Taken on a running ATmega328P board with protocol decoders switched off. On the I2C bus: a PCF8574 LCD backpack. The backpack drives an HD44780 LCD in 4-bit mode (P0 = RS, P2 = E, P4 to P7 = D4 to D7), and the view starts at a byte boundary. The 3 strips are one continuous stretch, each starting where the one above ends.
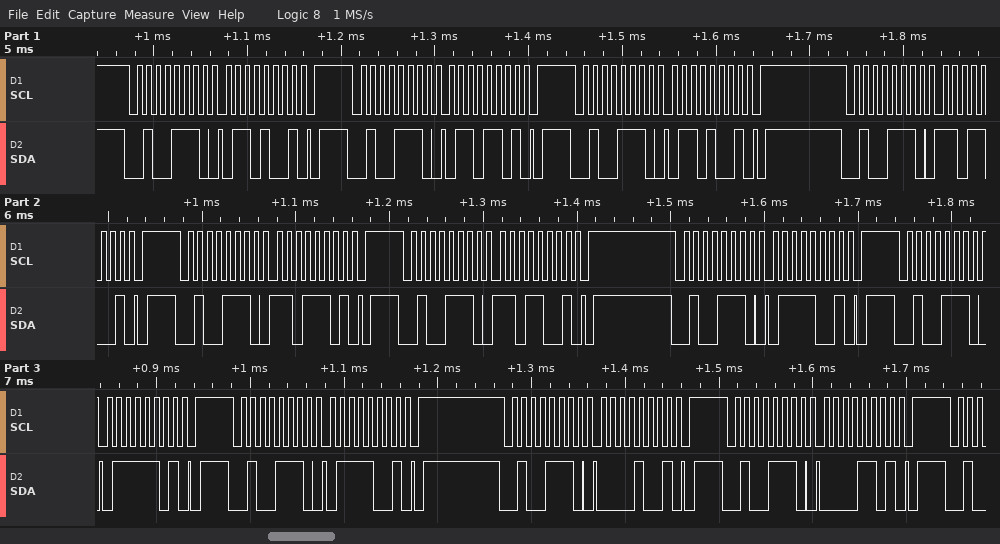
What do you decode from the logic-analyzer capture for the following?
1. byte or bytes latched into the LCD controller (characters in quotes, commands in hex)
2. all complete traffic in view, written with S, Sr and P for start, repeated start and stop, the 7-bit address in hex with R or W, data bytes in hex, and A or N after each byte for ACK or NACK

'm'
S 27W A 69 A P S 27W A 6D A P S 27W A 69 A P S 27W A D9 A P S 27W A DD A P S 27W A D9 A P S 27W A 79 A P S 27W A 7D A P S 27W A 79 A P S 27W A 09 A P S 27W A 0D A P
